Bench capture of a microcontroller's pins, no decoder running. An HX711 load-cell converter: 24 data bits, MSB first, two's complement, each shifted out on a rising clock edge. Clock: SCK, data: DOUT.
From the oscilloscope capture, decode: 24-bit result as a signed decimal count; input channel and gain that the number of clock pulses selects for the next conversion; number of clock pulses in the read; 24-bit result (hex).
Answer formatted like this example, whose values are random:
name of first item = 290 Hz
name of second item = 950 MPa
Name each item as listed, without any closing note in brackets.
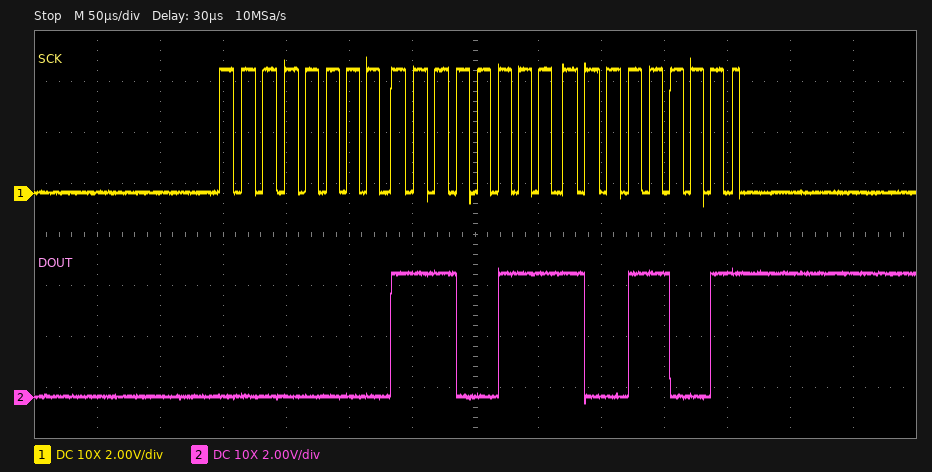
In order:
24-bit result as a signed decimal count = 59289
input channel and gain that the number of clock pulses selects for the next conversion = channel A, gain 128
number of clock pulses in the read = 25
24-bit result = 0x00E799
